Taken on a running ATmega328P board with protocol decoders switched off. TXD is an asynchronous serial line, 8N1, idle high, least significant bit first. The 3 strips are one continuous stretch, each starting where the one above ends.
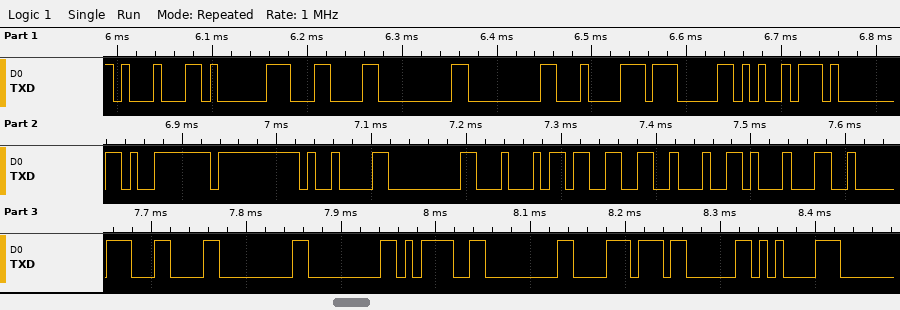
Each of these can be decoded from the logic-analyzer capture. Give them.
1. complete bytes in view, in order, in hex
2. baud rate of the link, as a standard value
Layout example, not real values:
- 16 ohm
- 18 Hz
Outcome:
- 11 81 0C 00 00 84 07 A5 01 F9 FF 09 00 44 33 22 11 82 0C 00 00 3D 00 B8 03 85
- 115200 baud
